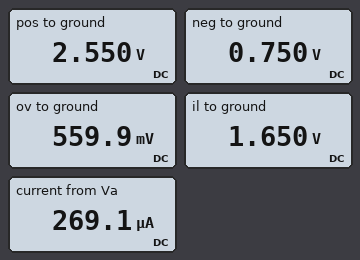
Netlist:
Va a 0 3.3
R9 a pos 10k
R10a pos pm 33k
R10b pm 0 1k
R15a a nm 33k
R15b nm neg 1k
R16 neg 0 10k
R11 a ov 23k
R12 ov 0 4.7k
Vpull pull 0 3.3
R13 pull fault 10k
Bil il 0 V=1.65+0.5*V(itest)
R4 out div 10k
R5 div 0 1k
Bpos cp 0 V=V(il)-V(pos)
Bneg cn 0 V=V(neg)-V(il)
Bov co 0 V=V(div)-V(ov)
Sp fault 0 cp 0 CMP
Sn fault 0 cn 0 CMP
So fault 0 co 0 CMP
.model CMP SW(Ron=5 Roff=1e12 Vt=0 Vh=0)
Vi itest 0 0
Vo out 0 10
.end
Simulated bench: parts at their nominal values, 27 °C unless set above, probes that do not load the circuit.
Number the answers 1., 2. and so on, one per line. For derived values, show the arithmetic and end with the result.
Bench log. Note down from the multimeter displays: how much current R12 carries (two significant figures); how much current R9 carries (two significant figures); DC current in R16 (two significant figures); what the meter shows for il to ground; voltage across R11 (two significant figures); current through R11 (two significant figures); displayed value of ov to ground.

1. (559.9 mV) / 4.7 kΩ = 120 µA
2. (3.3 V - 2.55 V) / 10 kΩ = 75 µA
3. (750 mV) / 10 kΩ = 75 µA
4. 1.650 V
5. 3.3 V - 559.9 mV = 2.7 V
6. (3.3 V - 559.9 mV) / 23 kΩ = 120 µA
7. 559.9 mV
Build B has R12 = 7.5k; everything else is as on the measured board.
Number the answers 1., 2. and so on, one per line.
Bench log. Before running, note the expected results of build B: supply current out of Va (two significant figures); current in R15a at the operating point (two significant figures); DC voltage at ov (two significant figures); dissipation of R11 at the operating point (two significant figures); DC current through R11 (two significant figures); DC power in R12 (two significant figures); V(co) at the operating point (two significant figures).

1. 260 µA
2. 75 µA
3. 810 mV
4. 270 µW
5. 110 µA
6. 88 µW
7. 98 mV
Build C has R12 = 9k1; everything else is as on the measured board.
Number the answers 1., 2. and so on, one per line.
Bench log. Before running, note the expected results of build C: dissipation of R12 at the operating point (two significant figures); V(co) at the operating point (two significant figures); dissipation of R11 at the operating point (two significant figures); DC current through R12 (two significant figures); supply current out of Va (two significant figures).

1. 96 µW
2. -26 mV
3. 240 µW
4. 100 µA
5. 250 µA
